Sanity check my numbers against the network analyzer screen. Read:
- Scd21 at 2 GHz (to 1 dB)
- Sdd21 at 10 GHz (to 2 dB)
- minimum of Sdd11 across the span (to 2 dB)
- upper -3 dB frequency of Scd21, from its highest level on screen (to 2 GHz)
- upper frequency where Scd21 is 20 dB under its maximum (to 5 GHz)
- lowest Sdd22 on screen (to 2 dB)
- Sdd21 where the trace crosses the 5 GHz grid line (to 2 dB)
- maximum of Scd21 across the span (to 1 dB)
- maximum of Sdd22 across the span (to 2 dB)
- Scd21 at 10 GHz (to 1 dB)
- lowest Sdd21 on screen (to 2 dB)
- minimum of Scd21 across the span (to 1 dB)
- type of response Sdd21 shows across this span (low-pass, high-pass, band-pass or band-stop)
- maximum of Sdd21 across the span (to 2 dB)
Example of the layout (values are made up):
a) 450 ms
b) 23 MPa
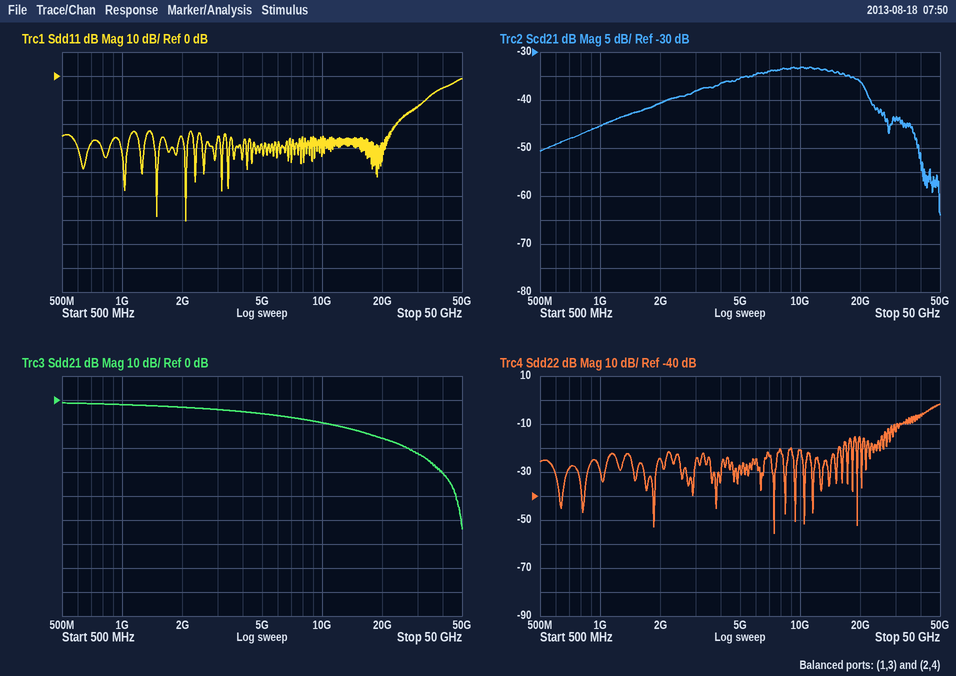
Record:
a) -41 dB
b) -10 dB
c) -60 dB
d) 20 GHz
e) 40 GHz
f) -56 dB
g) -6 dB
h) -33 dB
i) -2 dB
j) -33 dB
k) -54 dB
l) -64 dB
m) low-pass
n) -2 dB
